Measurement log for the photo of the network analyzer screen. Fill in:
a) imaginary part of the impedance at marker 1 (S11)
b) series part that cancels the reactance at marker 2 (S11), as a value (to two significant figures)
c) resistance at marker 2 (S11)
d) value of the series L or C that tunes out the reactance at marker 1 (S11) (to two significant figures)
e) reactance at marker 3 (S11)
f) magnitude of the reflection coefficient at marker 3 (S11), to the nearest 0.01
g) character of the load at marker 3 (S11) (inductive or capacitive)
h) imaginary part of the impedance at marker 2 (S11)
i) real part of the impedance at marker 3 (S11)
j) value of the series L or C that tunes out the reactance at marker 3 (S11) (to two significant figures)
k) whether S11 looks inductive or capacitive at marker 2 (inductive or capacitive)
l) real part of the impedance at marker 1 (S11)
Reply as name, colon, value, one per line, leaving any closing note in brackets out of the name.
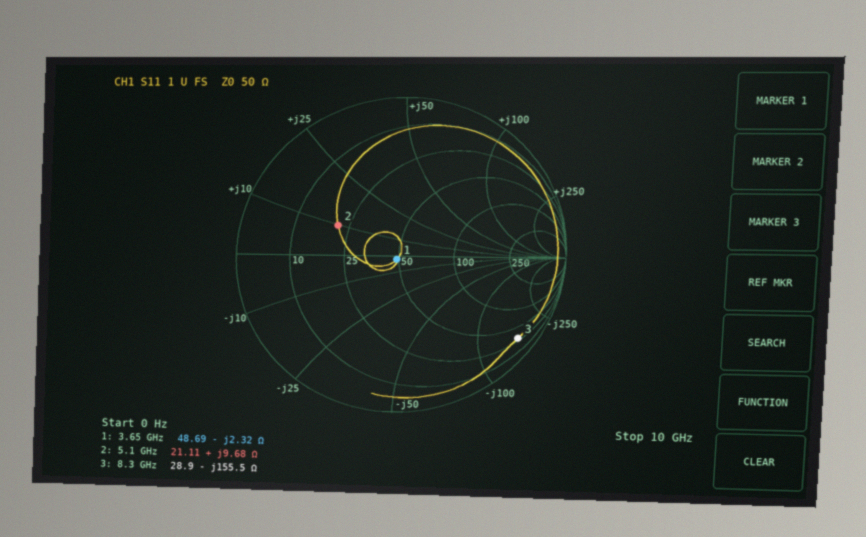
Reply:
imaginary part of the impedance at marker 1: -2.32 Ω
series part that cancels the reactance at marker 2 (S11), as a value: 3.2 pF
resistance at marker 2: 21.11 Ω
value of the series L or C that tunes out the reactance at marker 1 (S11): 100 pH
reactance at marker 3: -155.5 Ω
magnitude of the reflection coefficient at marker 3 (S11), to the nearest 0.01: 0.90
character of the load at marker 3 (S11): capacitive
imaginary part of the impedance at marker 2: +9.68 Ω
real part of the impedance at marker 3: 28.9 Ω
value of the series L or C that tunes out the reactance at marker 3 (S11): 3.0 nH
whether S11 looks inductive or capacitive at marker 2: inductive
real part of the impedance at marker 1: 48.69 Ω
